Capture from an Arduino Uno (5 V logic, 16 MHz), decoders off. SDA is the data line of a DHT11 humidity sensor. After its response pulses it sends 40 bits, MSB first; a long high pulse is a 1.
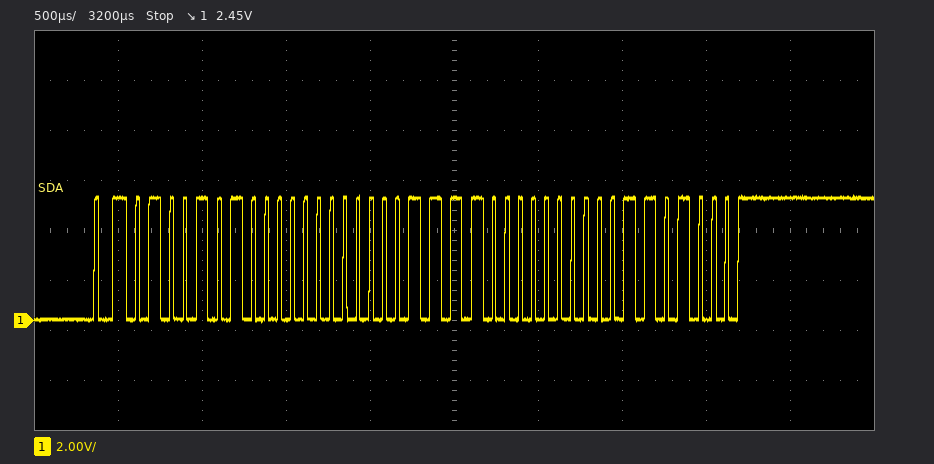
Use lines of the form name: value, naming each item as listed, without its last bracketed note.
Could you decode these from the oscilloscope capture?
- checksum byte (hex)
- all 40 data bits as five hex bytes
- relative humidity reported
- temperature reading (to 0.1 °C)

checksum byte: 0x68
all 40 data bits as five hex bytes: 4A 00 1E 00 68
relative humidity reported: 74 %
temperature reading: 30.0 °C
